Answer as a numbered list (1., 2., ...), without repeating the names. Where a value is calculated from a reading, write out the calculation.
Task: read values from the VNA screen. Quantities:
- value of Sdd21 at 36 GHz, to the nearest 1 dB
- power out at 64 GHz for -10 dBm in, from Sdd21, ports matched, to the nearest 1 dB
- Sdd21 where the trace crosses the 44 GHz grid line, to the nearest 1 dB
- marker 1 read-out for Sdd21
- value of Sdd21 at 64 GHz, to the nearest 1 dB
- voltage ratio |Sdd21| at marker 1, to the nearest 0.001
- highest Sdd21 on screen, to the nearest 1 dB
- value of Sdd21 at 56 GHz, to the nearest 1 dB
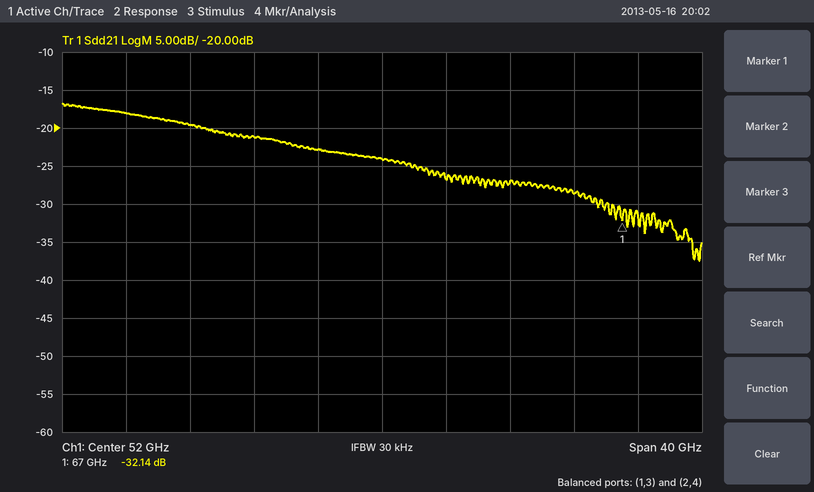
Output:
1. -18 dB
2. -10 dBm + (-29 dB) = -39 dBm
3. -21 dB
4. -32.14 dB
5. -29 dB
6. 10^(-32.14/20) ≈ 0.025
7. -17 dB
8. -27 dB
